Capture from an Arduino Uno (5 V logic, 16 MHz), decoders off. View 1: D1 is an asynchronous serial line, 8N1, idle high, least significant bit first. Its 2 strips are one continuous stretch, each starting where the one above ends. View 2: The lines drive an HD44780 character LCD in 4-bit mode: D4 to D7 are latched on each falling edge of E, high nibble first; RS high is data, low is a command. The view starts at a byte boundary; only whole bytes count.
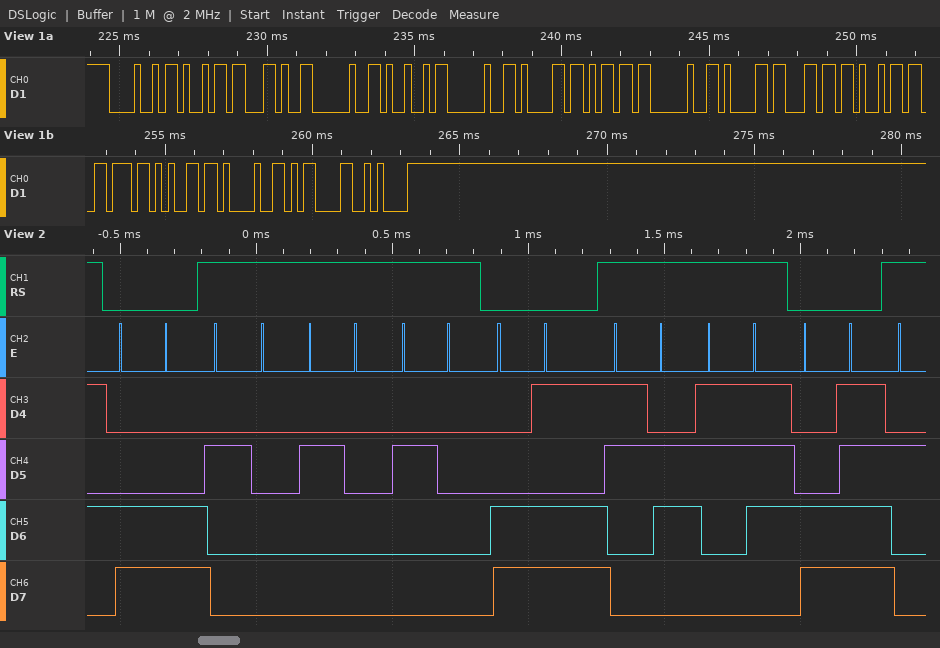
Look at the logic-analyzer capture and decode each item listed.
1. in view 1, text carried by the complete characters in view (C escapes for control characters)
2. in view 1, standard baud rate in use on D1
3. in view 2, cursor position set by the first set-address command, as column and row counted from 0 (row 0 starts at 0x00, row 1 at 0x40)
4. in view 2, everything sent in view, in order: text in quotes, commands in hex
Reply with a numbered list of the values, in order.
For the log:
1. "Hi, I am alive!\r\n"
2. 4800 baud
3. column 12, row 1
4. 0xCC "   " 0xCD "67" 0xCF
